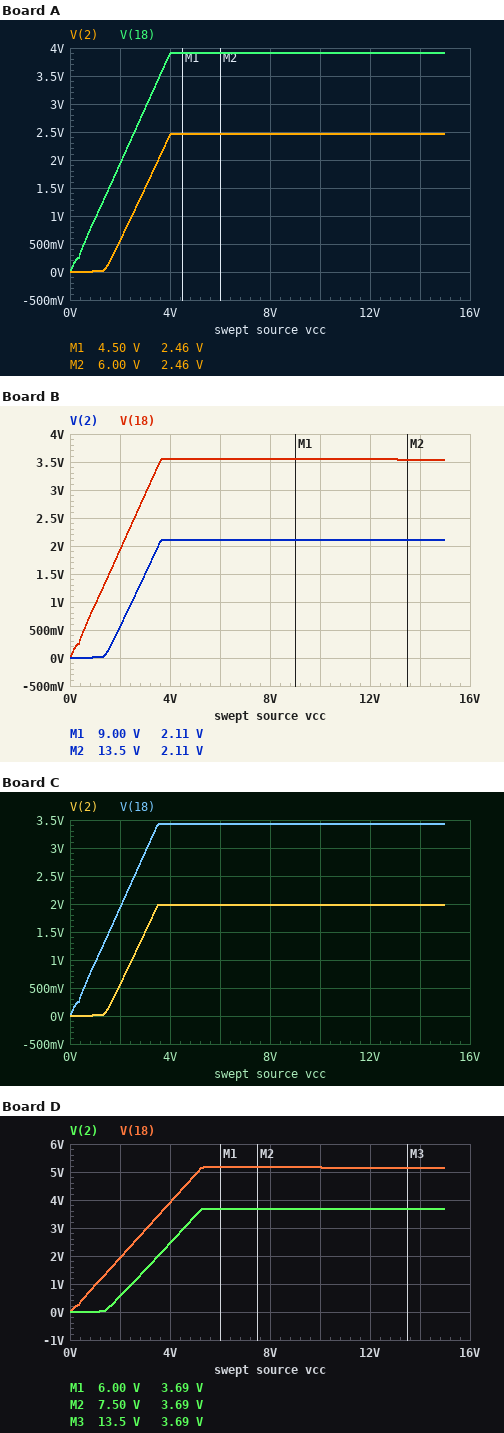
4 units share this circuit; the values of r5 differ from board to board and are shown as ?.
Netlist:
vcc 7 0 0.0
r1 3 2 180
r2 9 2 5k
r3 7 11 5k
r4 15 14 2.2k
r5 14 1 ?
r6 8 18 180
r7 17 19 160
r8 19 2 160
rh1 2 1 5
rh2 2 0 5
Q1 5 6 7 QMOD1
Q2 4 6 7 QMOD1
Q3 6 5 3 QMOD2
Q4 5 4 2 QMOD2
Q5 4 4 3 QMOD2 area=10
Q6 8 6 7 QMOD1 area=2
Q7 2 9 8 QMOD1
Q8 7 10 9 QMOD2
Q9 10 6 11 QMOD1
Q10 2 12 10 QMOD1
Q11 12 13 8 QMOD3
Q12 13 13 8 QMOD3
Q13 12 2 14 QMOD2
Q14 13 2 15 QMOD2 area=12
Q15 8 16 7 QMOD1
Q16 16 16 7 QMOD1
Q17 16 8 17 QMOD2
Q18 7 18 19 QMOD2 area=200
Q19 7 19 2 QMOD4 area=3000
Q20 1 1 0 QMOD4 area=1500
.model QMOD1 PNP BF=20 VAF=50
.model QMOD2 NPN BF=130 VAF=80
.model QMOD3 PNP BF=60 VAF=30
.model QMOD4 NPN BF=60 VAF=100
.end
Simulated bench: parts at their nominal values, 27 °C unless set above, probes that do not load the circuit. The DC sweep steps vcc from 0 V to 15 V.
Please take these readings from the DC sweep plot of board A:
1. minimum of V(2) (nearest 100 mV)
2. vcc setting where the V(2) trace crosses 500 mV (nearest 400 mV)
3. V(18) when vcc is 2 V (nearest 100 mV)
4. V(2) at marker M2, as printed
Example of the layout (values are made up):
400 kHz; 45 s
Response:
0 V; 2.0 V; 1.9 V; 2.46 V
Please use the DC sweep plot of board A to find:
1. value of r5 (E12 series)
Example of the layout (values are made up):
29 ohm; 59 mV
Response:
18 kΩ
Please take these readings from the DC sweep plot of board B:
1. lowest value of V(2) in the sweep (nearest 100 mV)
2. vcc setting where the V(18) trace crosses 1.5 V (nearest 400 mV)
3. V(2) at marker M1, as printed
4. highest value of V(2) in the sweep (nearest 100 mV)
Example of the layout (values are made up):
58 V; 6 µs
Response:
0 V; 1.6 V; 2.11 V; 2.1 V
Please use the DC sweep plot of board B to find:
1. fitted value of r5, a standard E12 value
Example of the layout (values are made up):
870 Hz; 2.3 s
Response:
12 kΩ
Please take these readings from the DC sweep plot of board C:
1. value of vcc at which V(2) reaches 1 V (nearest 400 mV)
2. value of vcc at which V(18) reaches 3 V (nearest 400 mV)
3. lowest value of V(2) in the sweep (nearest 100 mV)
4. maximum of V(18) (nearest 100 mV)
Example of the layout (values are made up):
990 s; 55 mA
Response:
2.4 V; 3.2 V; 0 V; 3.4 V
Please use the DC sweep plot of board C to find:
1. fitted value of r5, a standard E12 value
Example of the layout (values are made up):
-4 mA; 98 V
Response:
10 kΩ
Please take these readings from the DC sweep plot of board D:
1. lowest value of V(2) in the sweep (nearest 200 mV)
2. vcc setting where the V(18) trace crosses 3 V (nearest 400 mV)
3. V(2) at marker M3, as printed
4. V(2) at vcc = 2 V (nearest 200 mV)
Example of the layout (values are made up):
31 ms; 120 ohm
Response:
0 V; 3.2 V; 3.69 V; 600 mV
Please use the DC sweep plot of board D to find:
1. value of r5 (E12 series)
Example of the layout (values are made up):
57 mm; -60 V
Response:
39 kΩ
